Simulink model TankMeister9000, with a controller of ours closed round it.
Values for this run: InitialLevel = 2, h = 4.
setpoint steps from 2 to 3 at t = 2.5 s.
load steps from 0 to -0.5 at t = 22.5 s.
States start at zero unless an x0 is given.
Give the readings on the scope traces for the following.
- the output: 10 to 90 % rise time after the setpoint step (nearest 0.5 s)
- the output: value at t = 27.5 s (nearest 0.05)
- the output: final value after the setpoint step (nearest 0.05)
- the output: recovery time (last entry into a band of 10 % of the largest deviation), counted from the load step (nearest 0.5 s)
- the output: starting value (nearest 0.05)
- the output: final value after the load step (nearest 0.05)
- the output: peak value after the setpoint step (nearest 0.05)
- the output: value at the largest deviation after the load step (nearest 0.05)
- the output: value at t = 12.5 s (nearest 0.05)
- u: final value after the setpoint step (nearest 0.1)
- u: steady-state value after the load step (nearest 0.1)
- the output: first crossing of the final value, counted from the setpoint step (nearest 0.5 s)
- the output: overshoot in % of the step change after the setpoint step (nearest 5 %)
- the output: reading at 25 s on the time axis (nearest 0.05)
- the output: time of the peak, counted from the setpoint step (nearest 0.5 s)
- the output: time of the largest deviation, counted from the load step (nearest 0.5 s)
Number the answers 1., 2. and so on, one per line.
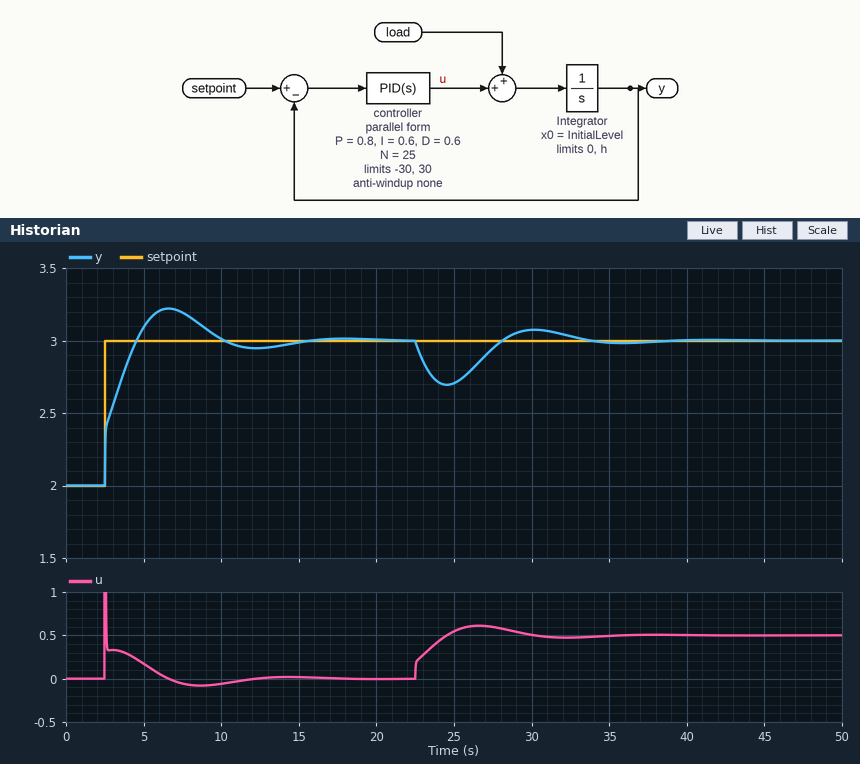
1. 1.5 s
2. 2.95
3. 3.00
4. 10.0 s
5. 2.00
6. 3.00
7. 3.20
8. 2.70
9. 2.95
10. 0.0
11. 0.5
12. 2.0 s
13. 20 %
14. 2.70
15. 4.0 s
16. 2.0 s
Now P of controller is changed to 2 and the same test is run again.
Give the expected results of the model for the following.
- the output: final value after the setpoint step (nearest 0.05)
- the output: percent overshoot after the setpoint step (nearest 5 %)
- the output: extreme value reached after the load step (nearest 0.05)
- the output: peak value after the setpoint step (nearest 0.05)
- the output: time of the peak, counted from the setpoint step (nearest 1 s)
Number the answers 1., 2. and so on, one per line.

1. 3.00
2. 10 %
3. 2.80
4. 3.10
5. 3 s
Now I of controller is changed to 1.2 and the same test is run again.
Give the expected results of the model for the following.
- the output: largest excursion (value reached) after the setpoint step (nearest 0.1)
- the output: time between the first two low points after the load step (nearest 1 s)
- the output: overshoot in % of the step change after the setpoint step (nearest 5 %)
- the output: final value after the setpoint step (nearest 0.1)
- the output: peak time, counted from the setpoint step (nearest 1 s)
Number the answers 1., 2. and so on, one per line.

1. 3.3
2. 8 s
3. 30 %
4. 3.0
5. 3 s
